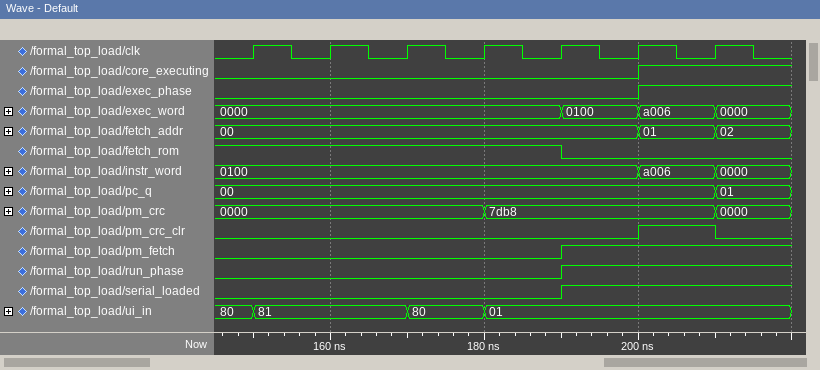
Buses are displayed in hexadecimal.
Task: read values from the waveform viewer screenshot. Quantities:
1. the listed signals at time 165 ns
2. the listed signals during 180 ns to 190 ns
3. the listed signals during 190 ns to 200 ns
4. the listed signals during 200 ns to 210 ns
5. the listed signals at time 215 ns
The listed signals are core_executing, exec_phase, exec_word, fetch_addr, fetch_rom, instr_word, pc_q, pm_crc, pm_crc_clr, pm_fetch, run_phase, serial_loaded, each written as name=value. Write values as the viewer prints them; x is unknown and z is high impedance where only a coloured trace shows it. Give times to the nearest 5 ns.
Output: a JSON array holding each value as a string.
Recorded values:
["core_executing=0, exec_phase=0, exec_word=0000, fetch_addr=00, fetch_rom=1, instr_word=0100, pc_q=00, pm_crc=0000, pm_crc_clr=0, pm_fetch=0, run_phase=0, serial_loaded=0", "core_executing=0, exec_phase=0, exec_word=0000, fetch_addr=00, fetch_rom=1, instr_word=0100, pc_q=00, pm_crc=7db8, pm_crc_clr=0, pm_fetch=0, run_phase=0, serial_loaded=0", "core_executing=0, exec_phase=0, exec_word=0100, fetch_addr=00, fetch_rom=0, instr_word=0100, pc_q=00, pm_crc=7db8, pm_crc_clr=0, pm_fetch=1, run_phase=1, serial_loaded=1", "core_executing=1, exec_phase=1, exec_word=a006, fetch_addr=01, fetch_rom=0, instr_word=a006, pc_q=00, pm_crc=7db8, pm_crc_clr=1, pm_fetch=1, run_phase=1, serial_loaded=1", "core_executing=1, exec_phase=1, exec_word=0000, fetch_addr=02, fetch_rom=0, instr_word=0000, pc_q=01, pm_crc=0000, pm_crc_clr=0, pm_fetch=1, run_phase=1, serial_loaded=1"]
